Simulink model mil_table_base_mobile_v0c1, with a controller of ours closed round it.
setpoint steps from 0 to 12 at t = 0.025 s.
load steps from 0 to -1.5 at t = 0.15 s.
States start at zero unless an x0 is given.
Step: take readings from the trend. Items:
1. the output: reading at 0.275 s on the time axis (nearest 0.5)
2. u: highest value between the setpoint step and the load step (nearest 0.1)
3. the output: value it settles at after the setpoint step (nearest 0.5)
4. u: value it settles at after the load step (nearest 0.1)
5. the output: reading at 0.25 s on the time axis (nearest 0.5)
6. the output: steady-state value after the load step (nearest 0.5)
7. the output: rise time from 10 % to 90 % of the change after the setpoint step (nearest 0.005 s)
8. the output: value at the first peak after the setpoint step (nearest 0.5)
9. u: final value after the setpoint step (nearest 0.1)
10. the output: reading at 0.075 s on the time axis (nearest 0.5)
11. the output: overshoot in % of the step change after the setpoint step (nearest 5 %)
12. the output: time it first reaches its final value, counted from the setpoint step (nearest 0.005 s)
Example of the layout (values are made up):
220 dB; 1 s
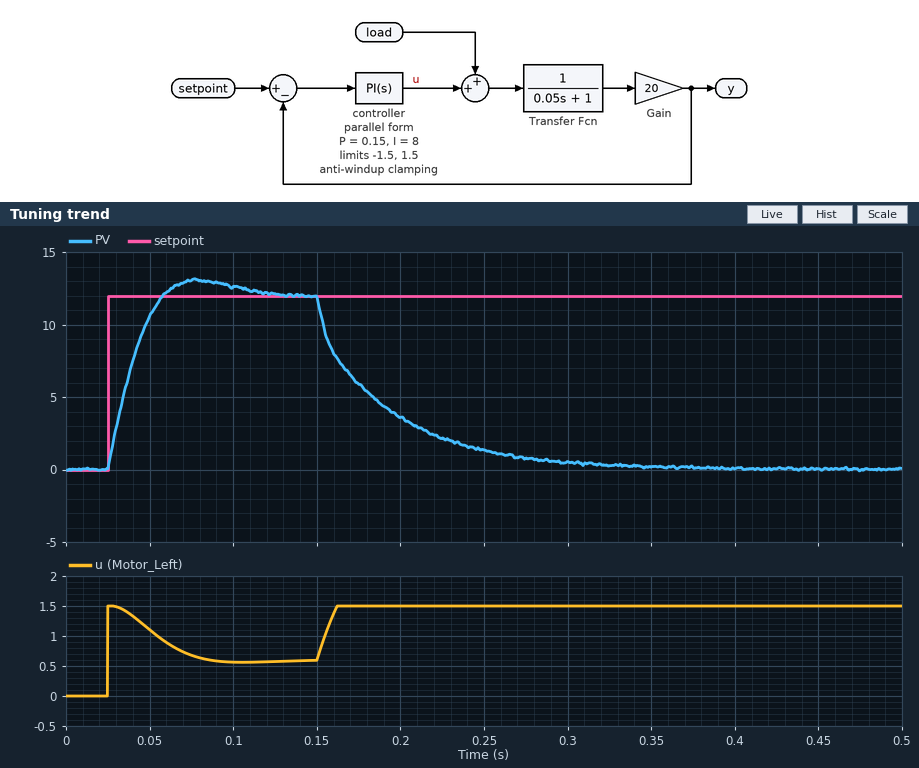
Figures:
1.0; 1.5; 12.0; 1.5; 1.5; 0.0; 0.025 s; 13.0; 0.6; 13.0; 10 %; 0.035 s
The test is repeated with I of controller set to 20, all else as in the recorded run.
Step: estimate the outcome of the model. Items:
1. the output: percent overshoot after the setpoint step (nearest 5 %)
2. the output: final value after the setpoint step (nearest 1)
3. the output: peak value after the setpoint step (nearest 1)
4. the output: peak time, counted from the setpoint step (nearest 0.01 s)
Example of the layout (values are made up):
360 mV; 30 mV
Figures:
15 %; 12; 14; 0.04 s
